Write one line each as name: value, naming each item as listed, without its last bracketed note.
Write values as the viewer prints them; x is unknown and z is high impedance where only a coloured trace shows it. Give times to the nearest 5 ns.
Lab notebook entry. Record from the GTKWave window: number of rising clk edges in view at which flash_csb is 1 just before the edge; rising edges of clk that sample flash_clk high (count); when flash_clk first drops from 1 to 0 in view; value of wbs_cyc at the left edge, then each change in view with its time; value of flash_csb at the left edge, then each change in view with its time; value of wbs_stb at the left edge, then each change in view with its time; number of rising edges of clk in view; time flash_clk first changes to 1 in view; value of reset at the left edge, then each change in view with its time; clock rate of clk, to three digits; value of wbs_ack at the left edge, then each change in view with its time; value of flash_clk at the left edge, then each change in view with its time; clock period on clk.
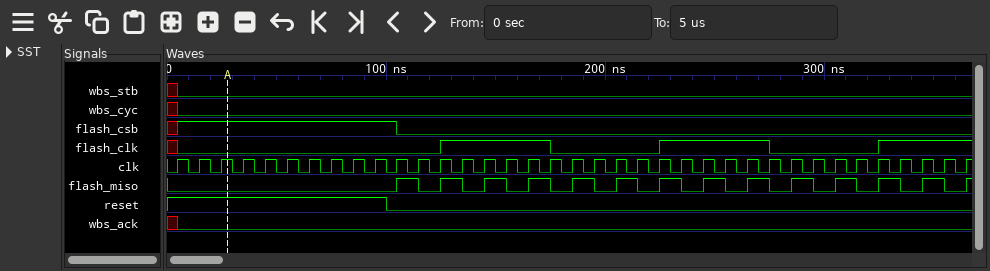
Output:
number of rising clk edges in view at which flash_csb is 1 just before the edge: 10
rising edges of clk that sample flash_clk high: 14
when flash_clk first drops from 1 to 0 in view: 175 ns
value of wbs_cyc at the left edge, then each change in view with its time: x, 0 at 5 ns
value of flash_csb at the left edge, then each change in view with its time: x, 1 at 5 ns, 0 at 105 ns
value of wbs_stb at the left edge, then each change in view with its time: x, 0 at 5 ns
number of rising edges of clk in view: 37
time flash_clk first changes to 1 in view: 125 ns
value of reset at the left edge, then each change in view with its time: 1, 0 at 100 ns
clock rate of clk, to three digits: 100 MHz
value of wbs_ack at the left edge, then each change in view with its time: x, 0 at 5 ns
value of flash_clk at the left edge, then each change in view with its time: x, 0 at 5 ns, 1 at 125 ns, 0 at 175 ns, 1 at 225 ns, 0 at 275 ns, 1 at 325 ns
clock period on clk: 10 ns
